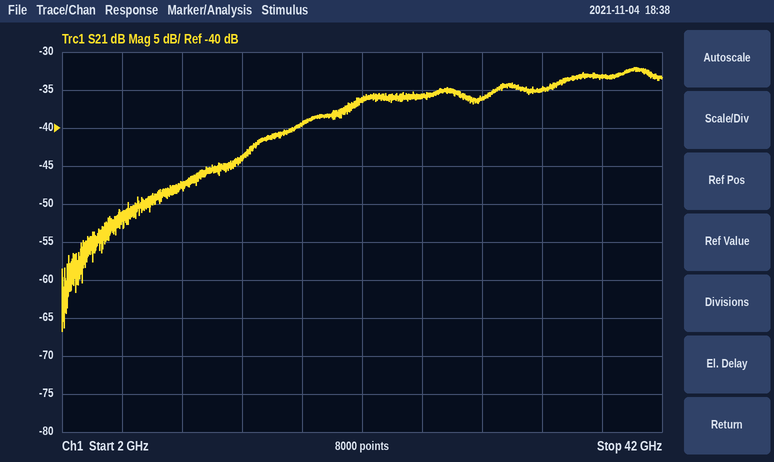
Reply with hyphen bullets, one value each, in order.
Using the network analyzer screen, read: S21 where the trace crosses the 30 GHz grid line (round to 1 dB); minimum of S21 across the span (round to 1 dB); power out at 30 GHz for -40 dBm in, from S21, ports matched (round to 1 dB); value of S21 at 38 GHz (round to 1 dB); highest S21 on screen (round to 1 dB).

- -36 dB
- -67 dB
- -76 dBm
- -33 dB
- -32 dB
